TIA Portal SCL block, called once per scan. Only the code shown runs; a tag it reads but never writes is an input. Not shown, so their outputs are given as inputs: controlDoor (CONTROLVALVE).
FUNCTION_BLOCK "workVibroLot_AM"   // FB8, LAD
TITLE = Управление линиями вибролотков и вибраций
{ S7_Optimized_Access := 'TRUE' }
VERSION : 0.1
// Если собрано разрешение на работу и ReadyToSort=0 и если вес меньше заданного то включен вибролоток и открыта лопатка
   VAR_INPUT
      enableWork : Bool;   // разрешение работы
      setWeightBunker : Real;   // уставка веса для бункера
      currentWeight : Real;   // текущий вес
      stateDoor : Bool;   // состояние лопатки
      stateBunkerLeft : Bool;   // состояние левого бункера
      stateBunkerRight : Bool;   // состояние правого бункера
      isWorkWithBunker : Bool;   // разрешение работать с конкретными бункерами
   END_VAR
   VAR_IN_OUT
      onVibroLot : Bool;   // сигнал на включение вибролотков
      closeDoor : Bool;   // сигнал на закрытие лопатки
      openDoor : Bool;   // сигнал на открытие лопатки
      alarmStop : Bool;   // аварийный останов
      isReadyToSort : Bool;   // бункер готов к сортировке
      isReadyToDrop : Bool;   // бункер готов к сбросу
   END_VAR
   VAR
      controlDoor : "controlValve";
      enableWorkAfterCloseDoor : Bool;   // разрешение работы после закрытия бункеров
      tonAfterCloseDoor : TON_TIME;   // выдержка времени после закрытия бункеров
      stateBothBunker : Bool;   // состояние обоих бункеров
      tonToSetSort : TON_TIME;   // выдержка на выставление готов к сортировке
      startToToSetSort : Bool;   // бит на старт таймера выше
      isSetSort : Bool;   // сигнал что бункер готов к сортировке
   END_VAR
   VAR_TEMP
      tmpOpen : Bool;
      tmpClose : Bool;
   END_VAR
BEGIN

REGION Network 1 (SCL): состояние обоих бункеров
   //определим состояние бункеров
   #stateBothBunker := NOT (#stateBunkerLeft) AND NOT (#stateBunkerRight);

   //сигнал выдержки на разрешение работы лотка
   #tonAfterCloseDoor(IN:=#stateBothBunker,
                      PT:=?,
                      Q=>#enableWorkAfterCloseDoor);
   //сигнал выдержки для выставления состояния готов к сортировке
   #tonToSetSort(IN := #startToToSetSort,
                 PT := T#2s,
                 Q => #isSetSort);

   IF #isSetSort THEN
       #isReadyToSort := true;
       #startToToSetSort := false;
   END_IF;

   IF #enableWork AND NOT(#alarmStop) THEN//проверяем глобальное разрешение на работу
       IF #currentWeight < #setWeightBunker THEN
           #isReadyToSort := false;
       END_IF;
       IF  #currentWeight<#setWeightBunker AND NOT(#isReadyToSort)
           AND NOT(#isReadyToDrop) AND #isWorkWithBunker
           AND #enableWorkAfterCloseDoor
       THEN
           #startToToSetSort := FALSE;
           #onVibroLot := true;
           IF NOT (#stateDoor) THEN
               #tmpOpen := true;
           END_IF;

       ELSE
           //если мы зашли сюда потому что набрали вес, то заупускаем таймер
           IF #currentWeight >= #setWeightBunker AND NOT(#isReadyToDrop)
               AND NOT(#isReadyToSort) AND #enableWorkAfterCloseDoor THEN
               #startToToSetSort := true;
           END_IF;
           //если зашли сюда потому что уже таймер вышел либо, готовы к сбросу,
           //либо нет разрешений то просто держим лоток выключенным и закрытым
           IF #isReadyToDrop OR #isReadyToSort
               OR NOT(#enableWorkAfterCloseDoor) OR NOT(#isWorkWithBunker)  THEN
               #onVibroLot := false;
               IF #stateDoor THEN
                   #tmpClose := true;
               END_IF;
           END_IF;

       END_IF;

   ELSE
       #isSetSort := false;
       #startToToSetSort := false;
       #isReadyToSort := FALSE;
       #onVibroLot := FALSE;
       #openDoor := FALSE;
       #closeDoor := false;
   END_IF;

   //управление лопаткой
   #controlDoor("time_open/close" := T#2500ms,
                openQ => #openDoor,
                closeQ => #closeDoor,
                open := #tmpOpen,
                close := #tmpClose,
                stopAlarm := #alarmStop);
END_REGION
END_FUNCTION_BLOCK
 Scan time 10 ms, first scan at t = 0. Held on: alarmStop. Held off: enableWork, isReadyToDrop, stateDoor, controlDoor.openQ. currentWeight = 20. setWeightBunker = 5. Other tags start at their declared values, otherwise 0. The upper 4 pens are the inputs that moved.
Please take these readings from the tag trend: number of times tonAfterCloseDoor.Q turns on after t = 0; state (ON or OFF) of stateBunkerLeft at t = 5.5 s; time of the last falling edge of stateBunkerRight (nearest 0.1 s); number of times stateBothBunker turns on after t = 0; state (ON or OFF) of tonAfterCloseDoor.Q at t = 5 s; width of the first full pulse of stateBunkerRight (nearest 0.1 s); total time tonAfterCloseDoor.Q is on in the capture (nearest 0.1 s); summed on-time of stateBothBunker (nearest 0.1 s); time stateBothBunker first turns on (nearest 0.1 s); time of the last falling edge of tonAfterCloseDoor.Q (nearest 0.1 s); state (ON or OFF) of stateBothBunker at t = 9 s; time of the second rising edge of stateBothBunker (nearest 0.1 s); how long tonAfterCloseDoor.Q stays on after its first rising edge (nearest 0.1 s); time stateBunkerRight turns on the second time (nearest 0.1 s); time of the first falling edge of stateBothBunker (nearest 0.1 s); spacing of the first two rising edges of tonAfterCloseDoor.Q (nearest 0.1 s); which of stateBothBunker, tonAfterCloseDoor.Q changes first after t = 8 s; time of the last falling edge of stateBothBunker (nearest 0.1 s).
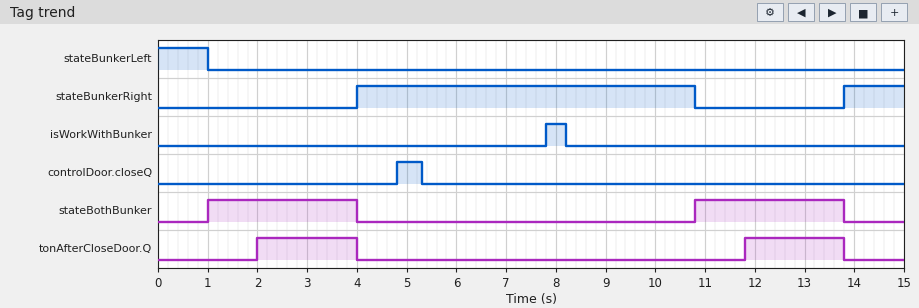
2
OFF
10.8 s
2
OFF
6.8 s
4.0 s
6.0 s
1.0 s
13.8 s
OFF
10.8 s
2.0 s
13.8 s
4.0 s
9.8 s
stateBothBunker
13.8 s
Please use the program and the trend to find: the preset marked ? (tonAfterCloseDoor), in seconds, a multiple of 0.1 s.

1.0 s
